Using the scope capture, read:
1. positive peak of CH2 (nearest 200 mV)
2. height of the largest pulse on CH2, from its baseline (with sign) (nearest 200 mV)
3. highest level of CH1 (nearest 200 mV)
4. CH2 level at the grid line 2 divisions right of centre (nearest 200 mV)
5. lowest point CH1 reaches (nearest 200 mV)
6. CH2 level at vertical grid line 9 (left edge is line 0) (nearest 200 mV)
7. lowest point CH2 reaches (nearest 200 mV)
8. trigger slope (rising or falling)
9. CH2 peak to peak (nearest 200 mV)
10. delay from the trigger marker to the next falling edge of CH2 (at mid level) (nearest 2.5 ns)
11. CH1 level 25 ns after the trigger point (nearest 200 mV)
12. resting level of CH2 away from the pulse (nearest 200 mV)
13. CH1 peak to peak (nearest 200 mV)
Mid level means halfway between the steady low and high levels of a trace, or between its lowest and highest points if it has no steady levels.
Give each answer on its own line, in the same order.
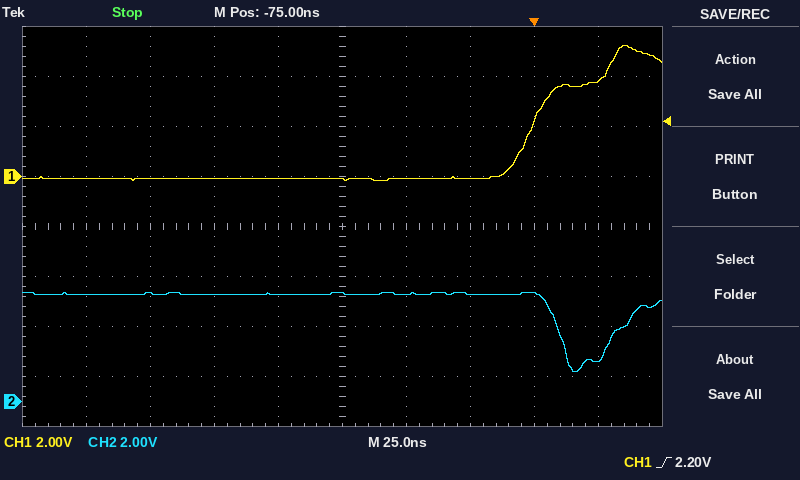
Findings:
4.4 V
-3.0 V
5.2 V
4.2 V
-200 mV
1.6 V
1.2 V
rising
3.2 V
10.0 ns
3.8 V
4.2 V
5.4 V
